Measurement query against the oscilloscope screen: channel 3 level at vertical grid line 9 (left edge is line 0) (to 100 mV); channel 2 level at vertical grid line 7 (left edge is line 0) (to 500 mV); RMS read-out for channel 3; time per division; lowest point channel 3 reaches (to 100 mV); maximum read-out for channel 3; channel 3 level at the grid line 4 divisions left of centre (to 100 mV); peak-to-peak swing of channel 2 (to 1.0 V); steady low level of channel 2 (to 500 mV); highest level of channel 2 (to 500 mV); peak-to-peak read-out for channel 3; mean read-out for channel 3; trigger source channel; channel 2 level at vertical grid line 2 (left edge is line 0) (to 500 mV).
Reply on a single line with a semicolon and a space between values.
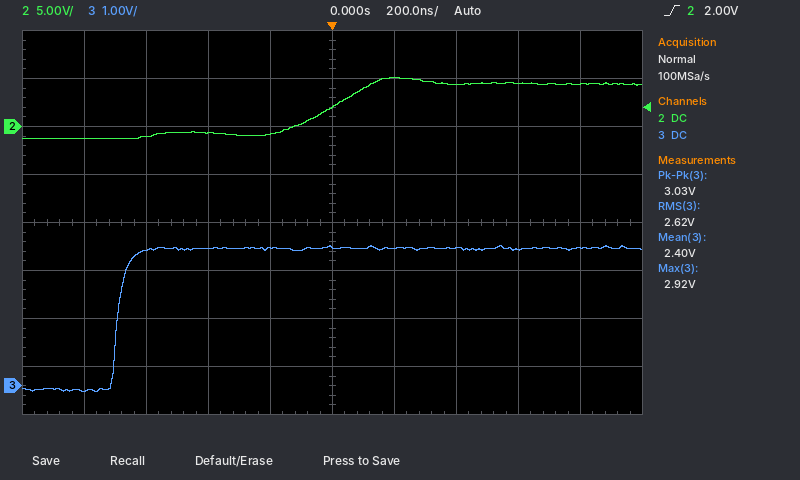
2.9 V; 4.5 V; 2.62 V; 200 ns; -100 mV; 2.92 V; -100 mV; 6.0 V; -1.0 V; 5.0 V; 3.03 V; 2.40 V; channel 2; -1.0 V
